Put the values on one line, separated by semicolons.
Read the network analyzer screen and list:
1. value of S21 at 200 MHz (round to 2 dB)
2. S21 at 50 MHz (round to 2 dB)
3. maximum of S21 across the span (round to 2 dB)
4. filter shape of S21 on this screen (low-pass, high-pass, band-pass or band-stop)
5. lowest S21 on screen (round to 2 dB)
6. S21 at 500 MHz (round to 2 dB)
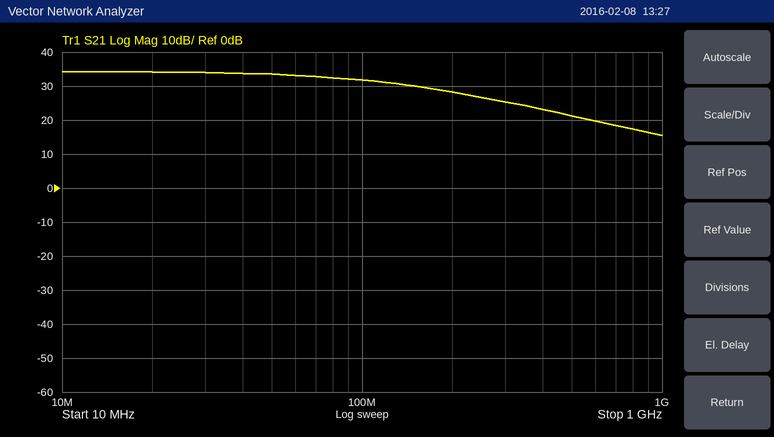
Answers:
28 dB; 34 dB; 34 dB; low-pass; 16 dB; 22 dB
